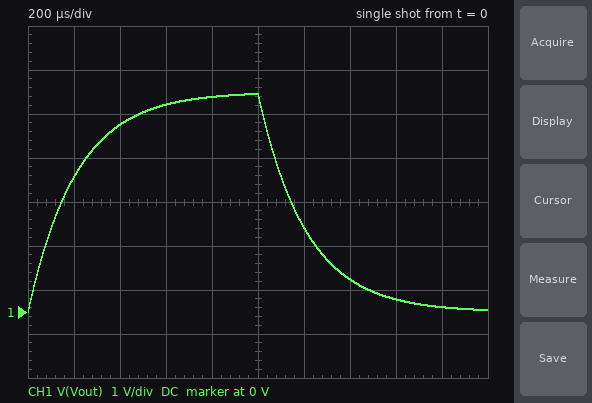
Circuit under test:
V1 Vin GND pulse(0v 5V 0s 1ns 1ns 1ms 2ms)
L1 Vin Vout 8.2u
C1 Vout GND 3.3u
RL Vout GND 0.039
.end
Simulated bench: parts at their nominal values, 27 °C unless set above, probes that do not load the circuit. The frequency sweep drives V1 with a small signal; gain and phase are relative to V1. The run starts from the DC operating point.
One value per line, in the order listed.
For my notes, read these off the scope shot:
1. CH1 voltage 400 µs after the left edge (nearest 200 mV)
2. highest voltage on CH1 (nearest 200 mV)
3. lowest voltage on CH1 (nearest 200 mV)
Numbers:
4.2 V
5.0 V
0 V
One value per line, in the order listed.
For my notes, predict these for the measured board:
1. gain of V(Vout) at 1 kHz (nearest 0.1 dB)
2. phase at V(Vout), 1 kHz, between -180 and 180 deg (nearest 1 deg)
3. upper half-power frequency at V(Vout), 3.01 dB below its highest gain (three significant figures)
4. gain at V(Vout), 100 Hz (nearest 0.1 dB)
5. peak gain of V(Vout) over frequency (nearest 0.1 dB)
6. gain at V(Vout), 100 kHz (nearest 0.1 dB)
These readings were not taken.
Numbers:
-4.4 dB
-53 deg
757 Hz
-0.1 dB
0 dB
-42.4 dB
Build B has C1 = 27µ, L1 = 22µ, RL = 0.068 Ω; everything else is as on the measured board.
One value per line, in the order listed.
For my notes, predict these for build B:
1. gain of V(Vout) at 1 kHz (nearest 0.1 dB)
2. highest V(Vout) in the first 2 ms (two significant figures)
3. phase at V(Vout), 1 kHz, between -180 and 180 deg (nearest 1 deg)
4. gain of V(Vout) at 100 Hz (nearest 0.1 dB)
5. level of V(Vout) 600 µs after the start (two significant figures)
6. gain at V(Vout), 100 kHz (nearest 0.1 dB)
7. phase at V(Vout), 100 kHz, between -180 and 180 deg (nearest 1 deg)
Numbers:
-7.1 dB
4.8 V
-64 deg
-0.2 dB
4.2 V
-49.8 dB
-139 deg
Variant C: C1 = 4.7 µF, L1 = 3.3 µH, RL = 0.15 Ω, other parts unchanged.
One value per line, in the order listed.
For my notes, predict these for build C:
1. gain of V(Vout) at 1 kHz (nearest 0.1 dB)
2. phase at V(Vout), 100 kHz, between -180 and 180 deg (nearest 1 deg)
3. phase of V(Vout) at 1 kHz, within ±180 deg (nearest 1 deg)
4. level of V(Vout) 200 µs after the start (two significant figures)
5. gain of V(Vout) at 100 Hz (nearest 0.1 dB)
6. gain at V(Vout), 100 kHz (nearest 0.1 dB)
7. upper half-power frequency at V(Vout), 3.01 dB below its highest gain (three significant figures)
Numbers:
-0.1 dB
-110 deg
-8 deg
5.0 V
0 dB
-23.4 dB
7.47 kHz
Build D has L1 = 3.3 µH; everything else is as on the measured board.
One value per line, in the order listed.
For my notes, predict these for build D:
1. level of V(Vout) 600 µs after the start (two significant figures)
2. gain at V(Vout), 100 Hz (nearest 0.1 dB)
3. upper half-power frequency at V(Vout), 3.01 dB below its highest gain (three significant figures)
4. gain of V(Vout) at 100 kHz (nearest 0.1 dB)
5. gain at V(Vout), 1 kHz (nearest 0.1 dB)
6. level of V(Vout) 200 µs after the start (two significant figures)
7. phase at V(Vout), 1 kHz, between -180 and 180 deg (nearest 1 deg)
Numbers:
5.0 V
0 dB
1.88 kHz
-34.5 dB
-1.1 dB
4.5 V
-28 deg
